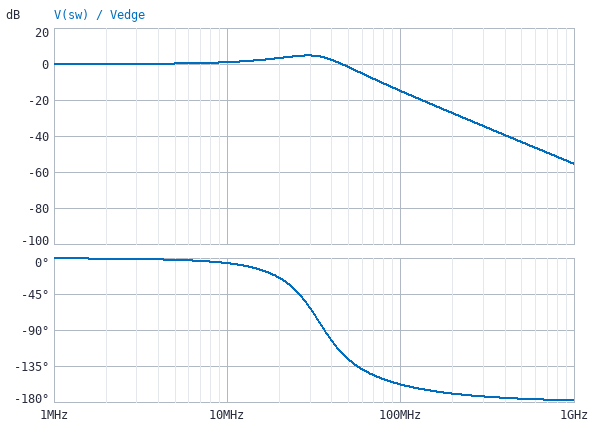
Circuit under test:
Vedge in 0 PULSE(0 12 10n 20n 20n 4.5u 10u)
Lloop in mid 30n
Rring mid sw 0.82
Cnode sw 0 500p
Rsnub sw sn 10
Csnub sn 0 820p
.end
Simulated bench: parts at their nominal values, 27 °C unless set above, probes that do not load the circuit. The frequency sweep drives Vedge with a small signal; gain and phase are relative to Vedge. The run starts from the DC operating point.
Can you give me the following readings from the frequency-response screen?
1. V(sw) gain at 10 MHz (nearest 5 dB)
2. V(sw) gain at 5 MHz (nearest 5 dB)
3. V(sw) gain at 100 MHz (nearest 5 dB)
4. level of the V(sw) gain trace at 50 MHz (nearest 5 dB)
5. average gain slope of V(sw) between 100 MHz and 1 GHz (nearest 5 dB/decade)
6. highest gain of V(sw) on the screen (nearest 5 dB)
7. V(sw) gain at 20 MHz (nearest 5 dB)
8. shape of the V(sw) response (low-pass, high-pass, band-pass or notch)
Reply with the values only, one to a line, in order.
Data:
0 dB
0 dB
-15 dB
0 dB
-40 dB/decade
5 dB
5 dB
low-pass
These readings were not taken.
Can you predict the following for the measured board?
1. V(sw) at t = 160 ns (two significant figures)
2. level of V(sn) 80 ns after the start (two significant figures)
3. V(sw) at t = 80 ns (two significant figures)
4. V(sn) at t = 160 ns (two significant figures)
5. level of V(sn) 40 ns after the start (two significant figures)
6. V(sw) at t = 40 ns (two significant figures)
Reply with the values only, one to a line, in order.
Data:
12 V
12 V
12 V
12 V
12 V
14 V
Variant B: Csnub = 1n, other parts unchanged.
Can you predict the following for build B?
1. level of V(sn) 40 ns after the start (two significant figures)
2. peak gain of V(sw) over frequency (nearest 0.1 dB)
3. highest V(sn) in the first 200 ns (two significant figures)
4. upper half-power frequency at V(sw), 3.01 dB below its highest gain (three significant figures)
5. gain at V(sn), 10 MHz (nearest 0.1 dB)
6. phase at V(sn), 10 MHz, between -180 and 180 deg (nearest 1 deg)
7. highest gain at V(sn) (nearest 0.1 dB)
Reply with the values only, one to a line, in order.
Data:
11 V
4.1 dB
12 V
42.7 MHz
-0.4 dB
-40 deg
0 dB
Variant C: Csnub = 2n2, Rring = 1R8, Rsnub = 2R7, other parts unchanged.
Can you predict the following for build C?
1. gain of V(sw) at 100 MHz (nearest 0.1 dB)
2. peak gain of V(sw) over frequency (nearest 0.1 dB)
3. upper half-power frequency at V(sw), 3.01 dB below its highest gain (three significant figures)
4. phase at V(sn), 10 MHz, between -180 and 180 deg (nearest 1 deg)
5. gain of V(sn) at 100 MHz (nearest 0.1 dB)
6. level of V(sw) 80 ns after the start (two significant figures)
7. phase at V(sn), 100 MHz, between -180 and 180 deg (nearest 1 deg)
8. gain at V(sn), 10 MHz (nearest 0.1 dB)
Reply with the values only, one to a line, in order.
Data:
-19.5 dB
1.5 dB
23.5 MHz
-45 deg
-31.2 dB
12 V
155 deg
0.6 dB
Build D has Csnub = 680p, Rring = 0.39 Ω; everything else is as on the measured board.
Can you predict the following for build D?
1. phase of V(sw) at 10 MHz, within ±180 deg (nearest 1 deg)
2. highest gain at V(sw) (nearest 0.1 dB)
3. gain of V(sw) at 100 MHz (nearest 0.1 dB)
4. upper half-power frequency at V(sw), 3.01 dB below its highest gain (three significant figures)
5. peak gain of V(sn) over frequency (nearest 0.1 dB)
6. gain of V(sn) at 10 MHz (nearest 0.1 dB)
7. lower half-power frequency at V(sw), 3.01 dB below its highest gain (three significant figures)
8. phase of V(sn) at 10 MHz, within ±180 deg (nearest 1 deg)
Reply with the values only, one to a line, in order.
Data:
-4 deg
6.7 dB
-15.0 dB
39.4 MHz
2.7 dB
0.4 dB
19.0 MHz
-27 deg
